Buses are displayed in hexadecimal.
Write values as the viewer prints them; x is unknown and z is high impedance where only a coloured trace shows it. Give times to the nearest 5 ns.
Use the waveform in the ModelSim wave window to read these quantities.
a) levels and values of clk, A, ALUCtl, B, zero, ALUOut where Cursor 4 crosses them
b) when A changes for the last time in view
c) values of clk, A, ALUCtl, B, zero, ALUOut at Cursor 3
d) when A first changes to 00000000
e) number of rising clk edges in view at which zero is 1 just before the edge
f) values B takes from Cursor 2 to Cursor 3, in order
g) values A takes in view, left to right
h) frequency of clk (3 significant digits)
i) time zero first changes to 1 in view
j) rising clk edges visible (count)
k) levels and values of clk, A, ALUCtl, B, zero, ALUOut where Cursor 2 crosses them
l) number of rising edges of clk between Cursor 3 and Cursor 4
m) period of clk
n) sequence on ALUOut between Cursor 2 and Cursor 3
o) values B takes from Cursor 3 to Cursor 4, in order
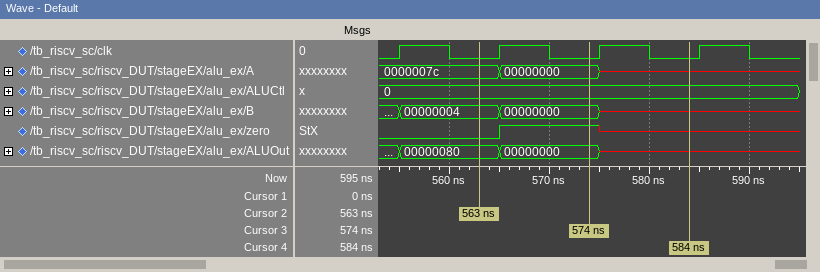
clk=0, A=x, ALUCtl=0, B=x, zero=x, ALUOut=x
575 ns
clk=0, A=00000000, ALUCtl=0, B=00000000, zero=1, ALUOut=00000000
565 ns
1
00000004, 00000000
0000007c, 00000000, x
100 MHz
565 ns
4
clk=0, A=0000007c, ALUCtl=0, B=00000004, zero=0, ALUOut=00000080
1
10 ns
00000080, 00000000
00000000, x
